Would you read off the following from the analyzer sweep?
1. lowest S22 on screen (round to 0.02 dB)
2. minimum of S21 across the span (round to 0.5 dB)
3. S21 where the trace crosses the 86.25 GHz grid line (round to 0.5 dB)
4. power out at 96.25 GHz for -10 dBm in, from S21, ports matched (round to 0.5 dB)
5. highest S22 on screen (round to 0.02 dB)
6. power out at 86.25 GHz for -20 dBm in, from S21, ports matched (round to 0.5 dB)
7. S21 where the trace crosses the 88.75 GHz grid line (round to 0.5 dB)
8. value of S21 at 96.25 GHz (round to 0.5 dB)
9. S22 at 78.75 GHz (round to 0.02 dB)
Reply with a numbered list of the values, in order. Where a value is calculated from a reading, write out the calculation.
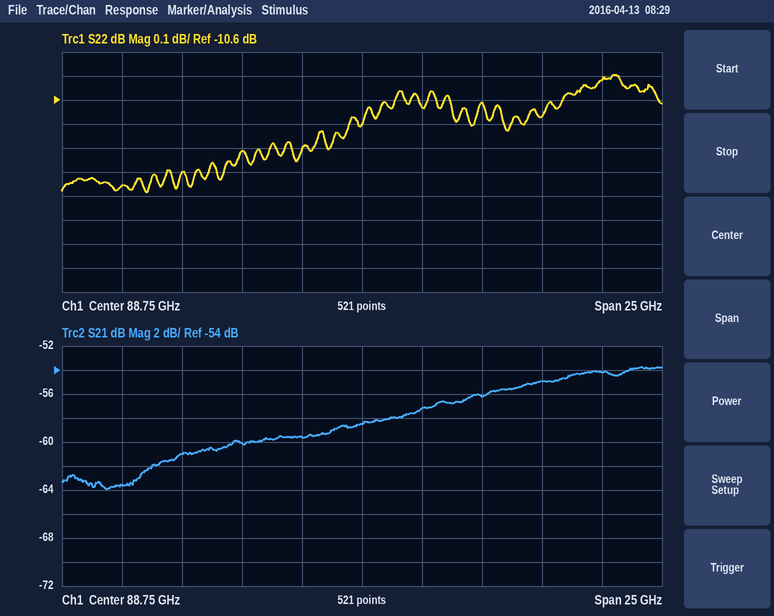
1. -10.98 dB
2. -64.0 dB
3. -59.5 dB
4. -10 dBm + (-55.0 dB) = -65.0 dBm
5. -10.50 dB
6. -20 dBm + (-59.5 dB) = -79.5 dBm
7. -58.5 dB
8. -55.0 dB
9. -10.96 dB
